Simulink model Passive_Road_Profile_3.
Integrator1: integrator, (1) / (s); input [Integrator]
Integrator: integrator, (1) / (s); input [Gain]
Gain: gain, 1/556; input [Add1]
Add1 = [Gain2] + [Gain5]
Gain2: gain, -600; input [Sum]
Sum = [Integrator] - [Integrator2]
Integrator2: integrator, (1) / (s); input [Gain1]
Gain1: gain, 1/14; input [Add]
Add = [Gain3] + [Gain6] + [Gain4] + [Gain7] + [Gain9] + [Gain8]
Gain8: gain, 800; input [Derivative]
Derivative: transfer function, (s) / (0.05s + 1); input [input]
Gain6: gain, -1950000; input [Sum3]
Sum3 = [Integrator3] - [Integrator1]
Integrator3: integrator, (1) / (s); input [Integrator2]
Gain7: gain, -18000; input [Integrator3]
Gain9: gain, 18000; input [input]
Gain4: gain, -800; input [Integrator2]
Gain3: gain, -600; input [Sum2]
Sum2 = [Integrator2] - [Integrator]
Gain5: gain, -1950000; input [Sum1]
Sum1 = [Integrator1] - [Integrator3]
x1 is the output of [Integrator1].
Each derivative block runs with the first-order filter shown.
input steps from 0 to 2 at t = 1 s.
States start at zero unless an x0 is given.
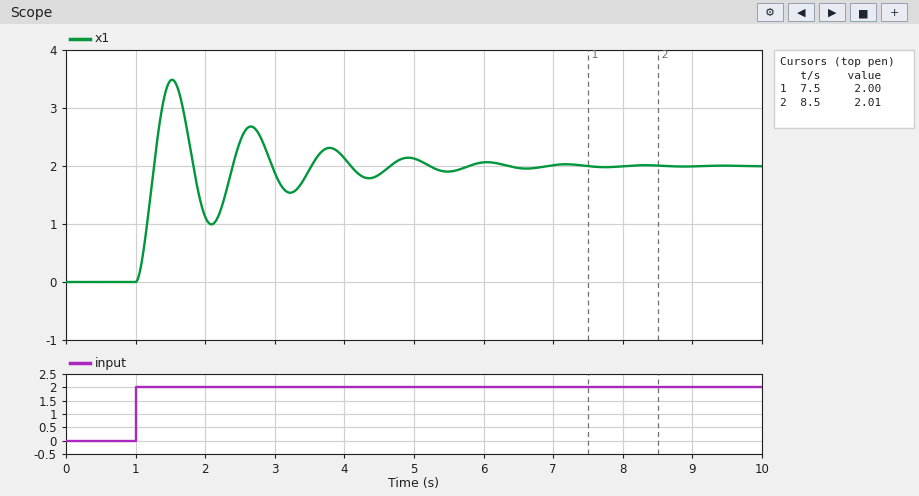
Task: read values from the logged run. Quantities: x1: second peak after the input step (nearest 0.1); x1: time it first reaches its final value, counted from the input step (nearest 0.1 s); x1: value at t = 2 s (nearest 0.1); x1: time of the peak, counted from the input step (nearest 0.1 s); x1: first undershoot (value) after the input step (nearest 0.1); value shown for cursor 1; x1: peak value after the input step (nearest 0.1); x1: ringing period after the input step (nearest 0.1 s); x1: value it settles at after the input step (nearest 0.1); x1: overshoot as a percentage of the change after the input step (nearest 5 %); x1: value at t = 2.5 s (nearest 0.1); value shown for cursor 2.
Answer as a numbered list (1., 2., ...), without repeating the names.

1. 2.7
2. 0.3 s
3. 1.1
4. 0.5 s
5. 1.0
6. 2.00
7. 3.5
8. 1.1 s
9. 2.0
10. 75 %
11. 2.4
12. 2.01
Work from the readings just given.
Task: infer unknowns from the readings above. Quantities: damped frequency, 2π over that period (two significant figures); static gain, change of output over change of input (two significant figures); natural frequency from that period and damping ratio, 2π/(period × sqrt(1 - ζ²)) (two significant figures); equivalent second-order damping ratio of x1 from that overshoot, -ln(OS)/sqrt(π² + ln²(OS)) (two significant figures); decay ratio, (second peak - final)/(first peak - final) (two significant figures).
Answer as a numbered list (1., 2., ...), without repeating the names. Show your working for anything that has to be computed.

1. 2π / 1.1 = 5.7 rad/s
2. (2 - 0) / (2 - 0) = 1.0
3. 2π / (1.1 × sqrt(1 - 0.091²)) = 5.7 rad/s
4. ln(0.75) = -0.288; 0.288 / sqrt(9.870 + 0.083) = 0.091
5. (2.7 - 2) / (3.5 - 2) = 0.47
